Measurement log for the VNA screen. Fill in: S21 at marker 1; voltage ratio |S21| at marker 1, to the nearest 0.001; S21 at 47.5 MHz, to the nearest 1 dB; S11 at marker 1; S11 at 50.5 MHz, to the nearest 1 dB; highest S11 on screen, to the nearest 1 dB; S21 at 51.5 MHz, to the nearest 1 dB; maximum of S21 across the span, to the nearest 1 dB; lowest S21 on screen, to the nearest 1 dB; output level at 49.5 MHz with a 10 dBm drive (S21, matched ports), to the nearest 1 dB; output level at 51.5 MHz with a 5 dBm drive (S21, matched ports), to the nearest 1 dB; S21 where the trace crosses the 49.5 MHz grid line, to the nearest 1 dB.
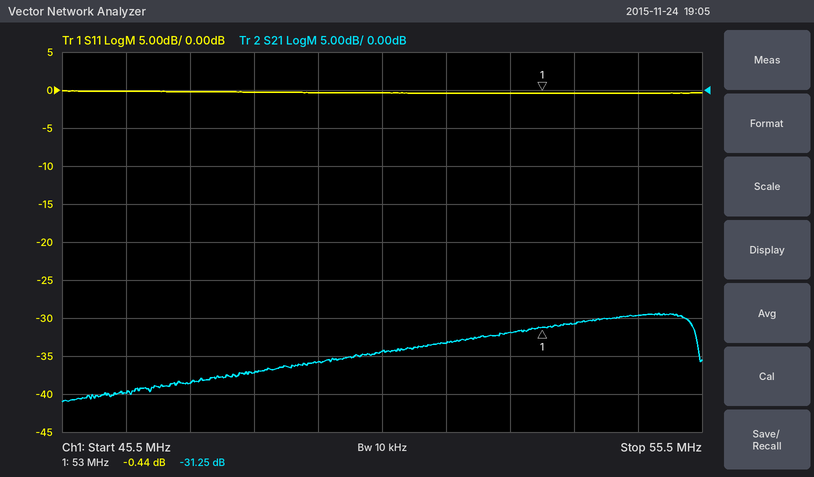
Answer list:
-31.25 dB
0.027
-39 dB
-0.44 dB
0 dB
0 dB
-33 dB
-29 dB
-41 dB
-26 dBm
-28 dBm
-36 dB
